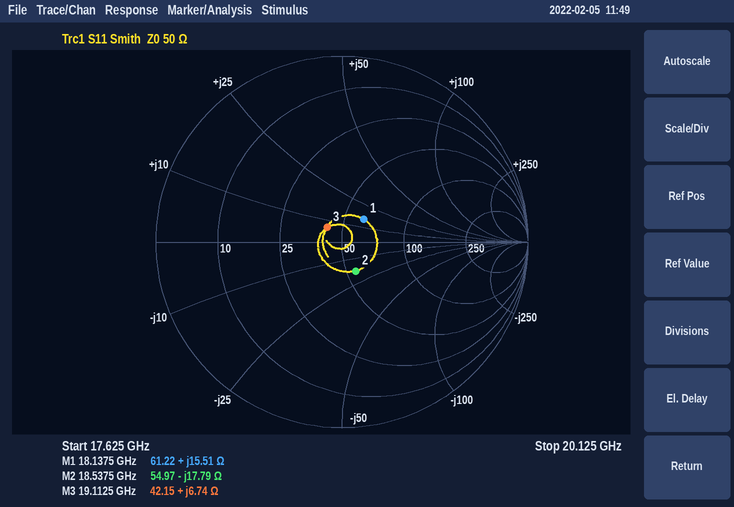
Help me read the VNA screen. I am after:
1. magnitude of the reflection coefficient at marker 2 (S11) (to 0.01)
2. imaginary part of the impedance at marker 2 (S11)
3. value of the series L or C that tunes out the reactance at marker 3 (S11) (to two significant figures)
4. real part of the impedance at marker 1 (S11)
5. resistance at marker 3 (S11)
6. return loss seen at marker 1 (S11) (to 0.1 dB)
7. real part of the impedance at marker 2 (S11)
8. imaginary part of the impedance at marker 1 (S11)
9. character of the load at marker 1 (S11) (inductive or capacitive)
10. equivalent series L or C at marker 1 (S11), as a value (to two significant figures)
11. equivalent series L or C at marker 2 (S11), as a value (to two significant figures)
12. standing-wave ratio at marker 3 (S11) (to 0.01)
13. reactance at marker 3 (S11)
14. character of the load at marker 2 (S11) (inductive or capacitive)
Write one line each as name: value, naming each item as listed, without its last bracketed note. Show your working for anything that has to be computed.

magnitude of the reflection coefficient at marker 2 (S11): 0.17
imaginary part of the impedance at marker 2: -17.79 Ω
value of the series L or C that tunes out the reactance at marker 3 (S11): C = 1/(2π × 19.1125 GHz × 6.74 Ω) ≈ 1.2 pF
real part of the impedance at marker 1: 61.22 Ω
resistance at marker 3: 42.15 Ω
return loss seen at marker 1 (S11): 15.4 dB
real part of the impedance at marker 2: 54.97 Ω
imaginary part of the impedance at marker 1: +15.51 Ω
character of the load at marker 1 (S11): inductive
equivalent series L or C at marker 1 (S11), as a value: L = 15.51 Ω/(2π × 18.1375 GHz) ≈ 136 pH, so 140 pH to two significant figures
equivalent series L or C at marker 2 (S11), as a value: C = 1/(2π × 18.5375 GHz × 17.79 Ω) ≈ 483 fF, so 480 fF to two significant figures
standing-wave ratio at marker 3 (S11): 1.25
reactance at marker 3: +6.74 Ω
character of the load at marker 2 (S11): capacitive
